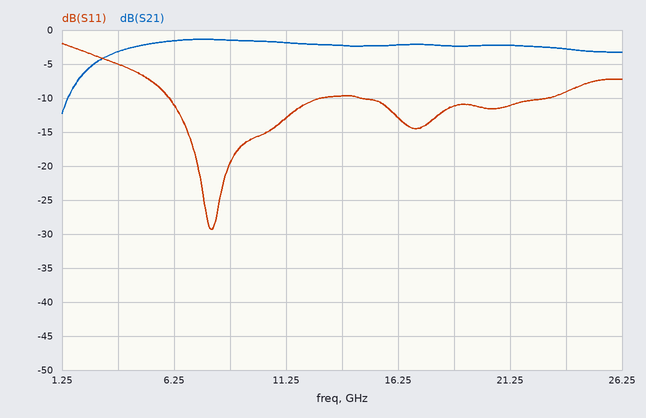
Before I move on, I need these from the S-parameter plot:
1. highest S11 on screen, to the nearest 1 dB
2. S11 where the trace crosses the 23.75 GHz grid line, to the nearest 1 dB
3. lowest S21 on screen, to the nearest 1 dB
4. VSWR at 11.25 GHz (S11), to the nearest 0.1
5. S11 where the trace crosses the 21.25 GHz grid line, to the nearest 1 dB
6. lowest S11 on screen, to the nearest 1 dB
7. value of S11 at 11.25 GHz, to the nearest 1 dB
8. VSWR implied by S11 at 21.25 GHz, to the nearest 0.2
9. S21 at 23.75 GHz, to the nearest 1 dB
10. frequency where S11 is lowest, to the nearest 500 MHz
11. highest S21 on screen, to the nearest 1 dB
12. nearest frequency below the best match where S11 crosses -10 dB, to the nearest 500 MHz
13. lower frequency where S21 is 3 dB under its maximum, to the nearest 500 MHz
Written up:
-2 dB
-9 dB
-12 dB
1.6
-11 dB
-29 dB
-13 dB
1.8
-3 dB
8.0 GHz
-1 dB
6.0 GHz
3.0 GHz
